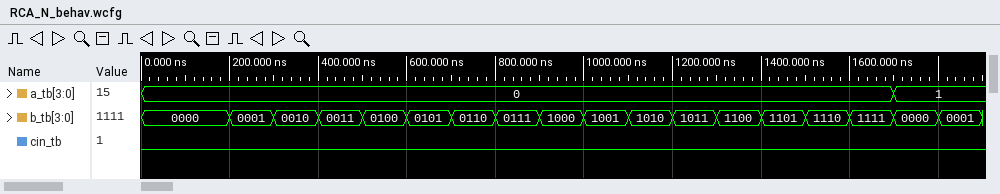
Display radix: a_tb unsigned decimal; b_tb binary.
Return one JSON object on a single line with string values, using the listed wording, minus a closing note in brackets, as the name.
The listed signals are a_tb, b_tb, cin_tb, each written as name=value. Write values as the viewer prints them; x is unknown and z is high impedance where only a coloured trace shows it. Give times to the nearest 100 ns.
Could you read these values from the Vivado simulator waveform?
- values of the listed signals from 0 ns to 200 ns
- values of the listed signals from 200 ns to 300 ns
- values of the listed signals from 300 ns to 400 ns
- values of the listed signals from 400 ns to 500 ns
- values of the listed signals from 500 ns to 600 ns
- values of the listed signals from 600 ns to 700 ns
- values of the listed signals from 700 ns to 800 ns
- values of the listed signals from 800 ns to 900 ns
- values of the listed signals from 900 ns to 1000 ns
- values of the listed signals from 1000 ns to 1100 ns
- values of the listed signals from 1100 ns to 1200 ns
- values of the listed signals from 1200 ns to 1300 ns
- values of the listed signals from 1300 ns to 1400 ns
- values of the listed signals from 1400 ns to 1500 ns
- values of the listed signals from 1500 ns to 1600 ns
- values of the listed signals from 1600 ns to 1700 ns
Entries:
{"values of the listed signals from 0 ns to 200 ns": "a_tb=0, b_tb=0000, cin_tb=0", "values of the listed signals from 200 ns to 300 ns": "a_tb=0, b_tb=0001, cin_tb=0", "values of the listed signals from 300 ns to 400 ns": "a_tb=0, b_tb=0010, cin_tb=0", "values of the listed signals from 400 ns to 500 ns": "a_tb=0, b_tb=0011, cin_tb=0", "values of the listed signals from 500 ns to 600 ns": "a_tb=0, b_tb=0100, cin_tb=0", "values of the listed signals from 600 ns to 700 ns": "a_tb=0, b_tb=0101, cin_tb=0", "values of the listed signals from 700 ns to 800 ns": "a_tb=0, b_tb=0110, cin_tb=0", "values of the listed signals from 800 ns to 900 ns": "a_tb=0, b_tb=0111, cin_tb=0", "values of the listed signals from 900 ns to 1000 ns": "a_tb=0, b_tb=1000, cin_tb=0", "values of the listed signals from 1000 ns to 1100 ns": "a_tb=0, b_tb=1001, cin_tb=0", "values of the listed signals from 1100 ns to 1200 ns": "a_tb=0, b_tb=1010, cin_tb=0", "values of the listed signals from 1200 ns to 1300 ns": "a_tb=0, b_tb=1011, cin_tb=0", "values of the listed signals from 1300 ns to 1400 ns": "a_tb=0, b_tb=1100, cin_tb=0", "values of the listed signals from 1400 ns to 1500 ns": "a_tb=0, b_tb=1101, cin_tb=0", "values of the listed signals from 1500 ns to 1600 ns": "a_tb=0, b_tb=1110, cin_tb=0", "values of the listed signals from 1600 ns to 1700 ns": "a_tb=0, b_tb=1111, cin_tb=0"}
